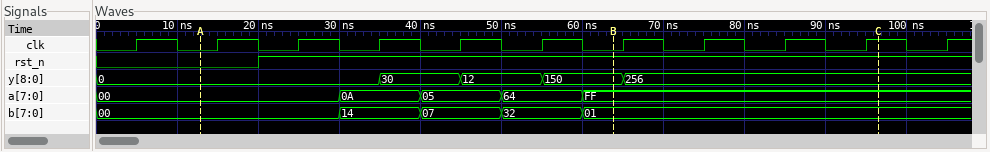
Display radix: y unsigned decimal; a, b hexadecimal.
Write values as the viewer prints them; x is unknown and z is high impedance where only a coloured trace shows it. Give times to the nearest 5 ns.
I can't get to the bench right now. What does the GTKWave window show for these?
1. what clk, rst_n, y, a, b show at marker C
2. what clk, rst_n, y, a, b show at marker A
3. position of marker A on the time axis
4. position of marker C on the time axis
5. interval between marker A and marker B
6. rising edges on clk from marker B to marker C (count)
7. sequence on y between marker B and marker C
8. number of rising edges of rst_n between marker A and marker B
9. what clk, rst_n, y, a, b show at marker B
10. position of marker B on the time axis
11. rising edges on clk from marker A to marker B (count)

clk=1, rst_n=1, y=256, a=FF, b=01
clk=0, rst_n=0, y=0, a=00, b=00
15 ns
95 ns
50 ns
4
150, 256
1
clk=0, rst_n=1, y=150, a=FF, b=01
65 ns
5
